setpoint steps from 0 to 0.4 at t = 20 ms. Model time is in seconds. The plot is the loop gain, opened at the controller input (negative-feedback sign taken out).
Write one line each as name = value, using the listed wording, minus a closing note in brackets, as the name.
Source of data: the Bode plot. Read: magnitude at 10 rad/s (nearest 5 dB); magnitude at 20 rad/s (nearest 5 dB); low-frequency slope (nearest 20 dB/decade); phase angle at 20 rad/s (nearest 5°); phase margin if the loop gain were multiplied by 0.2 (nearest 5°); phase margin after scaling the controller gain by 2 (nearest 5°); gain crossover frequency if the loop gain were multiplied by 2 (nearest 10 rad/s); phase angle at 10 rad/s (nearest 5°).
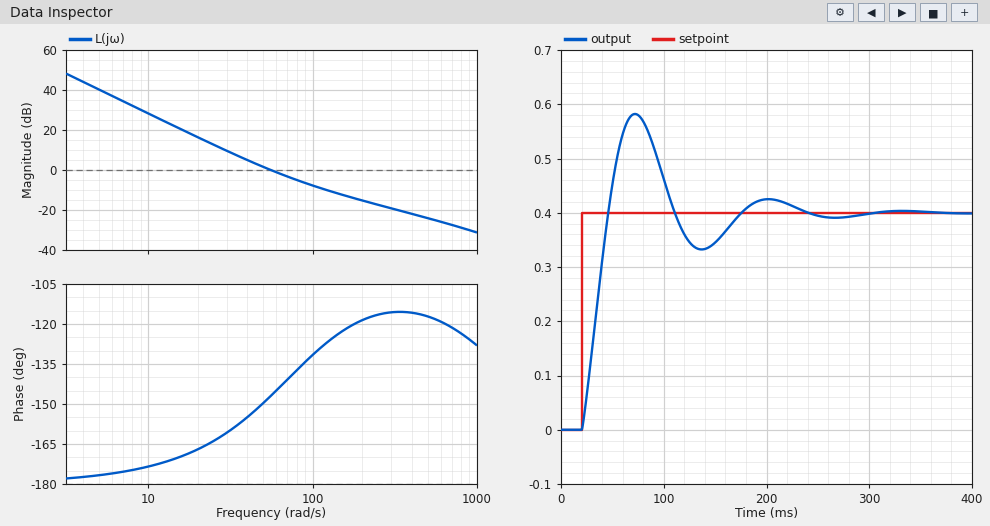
magnitude at 10 rad/s = 30 dB
magnitude at 20 rad/s = 15 dB
low-frequency slope = -40 dB/decade
phase angle at 20 rad/s = -165°
phase margin if the loop gain were multiplied by 0.2 = 15°
phase margin after scaling the controller gain by 2 = 45°
gain crossover frequency if the loop gain were multiplied by 2 = 90 rad/s
phase angle at 10 rad/s = -175°
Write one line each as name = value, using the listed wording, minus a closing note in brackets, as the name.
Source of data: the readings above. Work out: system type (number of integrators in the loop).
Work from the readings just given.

system type = 2
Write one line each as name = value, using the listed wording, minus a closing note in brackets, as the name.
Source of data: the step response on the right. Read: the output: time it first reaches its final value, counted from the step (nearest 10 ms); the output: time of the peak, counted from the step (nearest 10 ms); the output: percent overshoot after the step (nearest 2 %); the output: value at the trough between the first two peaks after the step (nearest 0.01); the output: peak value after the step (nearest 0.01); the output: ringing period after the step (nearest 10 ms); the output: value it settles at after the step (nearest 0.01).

the output: time it first reaches its final value, counted from the step = 30 ms
the output: time of the peak, counted from the step = 50 ms
the output: percent overshoot after the step = 46 %
the output: value at the trough between the first two peaks after the step = 0.33
the output: peak value after the step = 0.58
the output: ringing period after the step = 130 ms
the output: value it settles at after the step = 0.40
